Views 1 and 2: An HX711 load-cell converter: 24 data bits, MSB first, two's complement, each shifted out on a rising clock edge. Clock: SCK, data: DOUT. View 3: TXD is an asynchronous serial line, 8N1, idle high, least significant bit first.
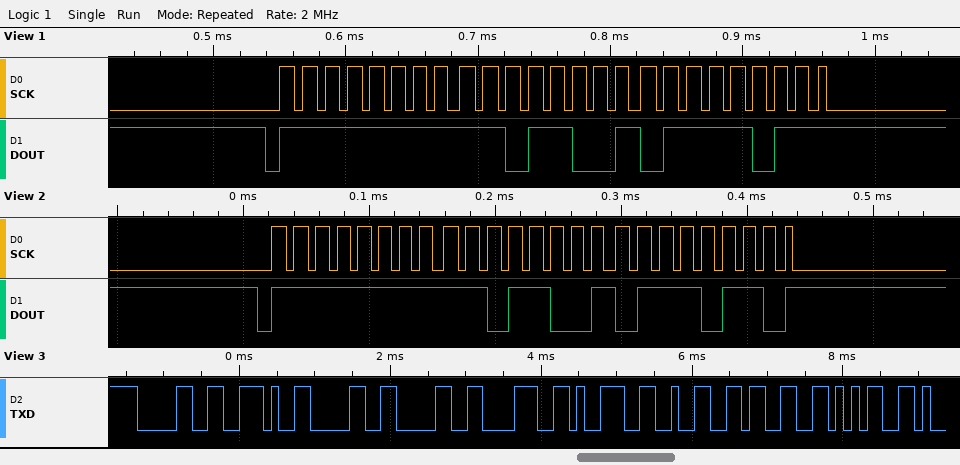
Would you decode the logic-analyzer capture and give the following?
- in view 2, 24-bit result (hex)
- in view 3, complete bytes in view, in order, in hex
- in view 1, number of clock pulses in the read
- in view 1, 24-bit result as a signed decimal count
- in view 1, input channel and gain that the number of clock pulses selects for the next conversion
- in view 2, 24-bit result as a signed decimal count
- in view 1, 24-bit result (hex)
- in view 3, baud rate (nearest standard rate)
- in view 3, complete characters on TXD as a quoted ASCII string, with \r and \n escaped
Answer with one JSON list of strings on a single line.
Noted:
["0xFFD976", "0x30 0x2E 0x30 0x30 0x38 0x39 0x32 0x33 0x35", "25", "-9861", "channel A, gain 128", "-9866", "0xFFD97B", "9600 baud", "\"0.0089235\""]
